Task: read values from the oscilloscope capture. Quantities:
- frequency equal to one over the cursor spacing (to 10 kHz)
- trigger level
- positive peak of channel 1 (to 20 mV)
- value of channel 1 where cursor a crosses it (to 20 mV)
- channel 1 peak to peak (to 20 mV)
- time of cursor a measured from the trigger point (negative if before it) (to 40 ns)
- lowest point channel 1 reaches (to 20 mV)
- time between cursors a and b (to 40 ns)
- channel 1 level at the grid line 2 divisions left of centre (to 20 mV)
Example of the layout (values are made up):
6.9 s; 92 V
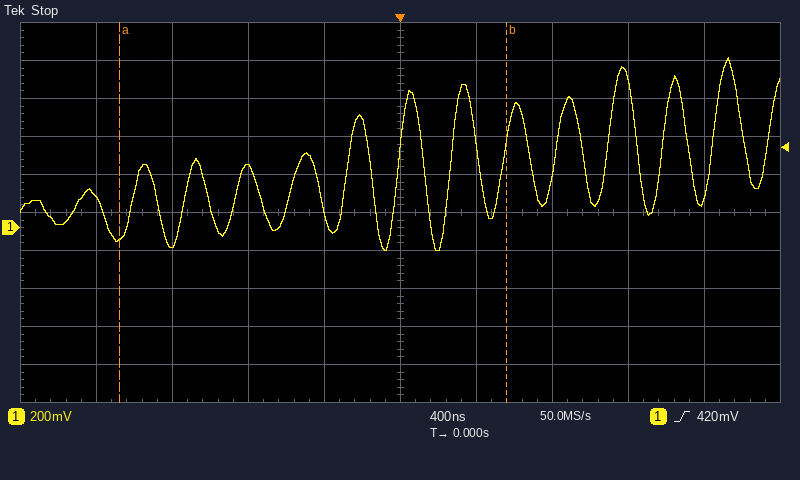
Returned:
490 kHz; 420 mV; 900 mV; -60 mV; 1.02 V; -1.48 µs; -120 mV; 2.04 µs; 320 mV
